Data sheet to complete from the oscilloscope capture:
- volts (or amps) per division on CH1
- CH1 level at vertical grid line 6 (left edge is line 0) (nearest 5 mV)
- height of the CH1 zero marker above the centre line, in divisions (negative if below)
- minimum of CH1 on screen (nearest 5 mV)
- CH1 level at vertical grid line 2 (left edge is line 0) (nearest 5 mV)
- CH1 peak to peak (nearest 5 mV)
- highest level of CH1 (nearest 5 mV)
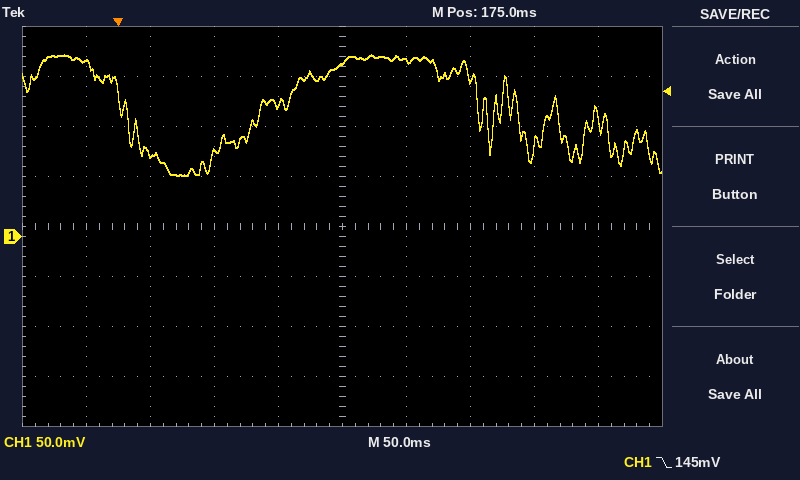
50 mV
175 mV
-0.2 div
60 mV
85 mV
120 mV
180 mV
